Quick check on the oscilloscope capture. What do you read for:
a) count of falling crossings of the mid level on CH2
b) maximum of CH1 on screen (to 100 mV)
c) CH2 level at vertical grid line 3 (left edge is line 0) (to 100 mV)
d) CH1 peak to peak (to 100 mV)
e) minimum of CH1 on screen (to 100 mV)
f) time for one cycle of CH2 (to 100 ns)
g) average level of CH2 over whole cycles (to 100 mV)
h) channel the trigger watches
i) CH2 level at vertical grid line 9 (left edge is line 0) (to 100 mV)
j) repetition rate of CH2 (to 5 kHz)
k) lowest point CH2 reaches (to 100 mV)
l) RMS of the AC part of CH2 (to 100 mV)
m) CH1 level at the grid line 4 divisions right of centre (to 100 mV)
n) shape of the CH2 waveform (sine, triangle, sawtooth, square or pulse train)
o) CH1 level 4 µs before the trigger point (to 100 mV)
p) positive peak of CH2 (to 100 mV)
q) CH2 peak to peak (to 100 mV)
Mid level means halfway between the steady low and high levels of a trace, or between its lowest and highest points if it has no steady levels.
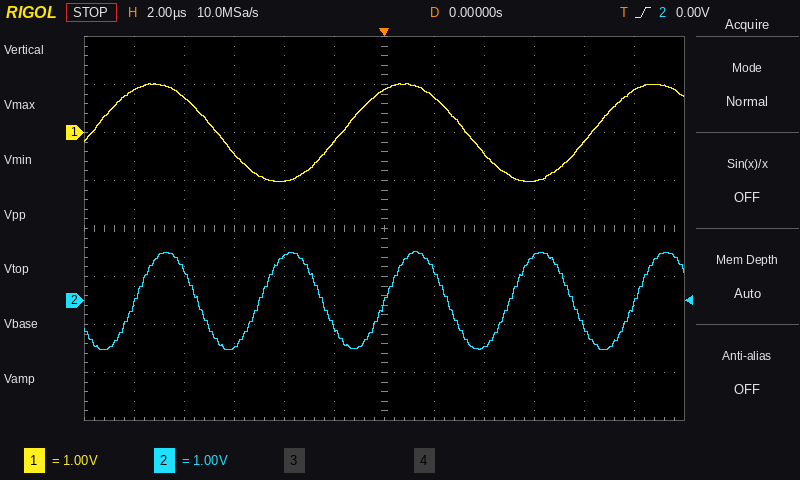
4
1.0 V
-1.0 V
2.0 V
-1.0 V
5.0 µs
0.0 V
CH2
900 mV
200 kHz
-1.0 V
700 mV
-200 mV
sine
-1.0 V
1.0 V
2.0 V
